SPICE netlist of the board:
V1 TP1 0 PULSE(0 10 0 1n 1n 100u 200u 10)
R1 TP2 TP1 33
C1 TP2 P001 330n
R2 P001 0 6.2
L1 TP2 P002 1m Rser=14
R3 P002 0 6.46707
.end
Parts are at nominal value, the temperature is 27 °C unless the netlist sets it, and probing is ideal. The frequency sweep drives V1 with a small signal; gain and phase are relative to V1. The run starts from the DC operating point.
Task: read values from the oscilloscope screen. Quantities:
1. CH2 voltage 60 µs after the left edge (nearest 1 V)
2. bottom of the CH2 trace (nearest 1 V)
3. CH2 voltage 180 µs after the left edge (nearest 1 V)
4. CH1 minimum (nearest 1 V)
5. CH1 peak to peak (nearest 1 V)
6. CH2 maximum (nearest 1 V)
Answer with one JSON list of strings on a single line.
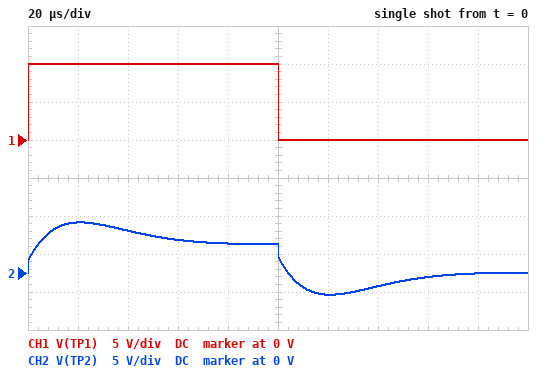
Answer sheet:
["4 V", "-3 V", "0 V", "0 V", "10 V", "7 V"]
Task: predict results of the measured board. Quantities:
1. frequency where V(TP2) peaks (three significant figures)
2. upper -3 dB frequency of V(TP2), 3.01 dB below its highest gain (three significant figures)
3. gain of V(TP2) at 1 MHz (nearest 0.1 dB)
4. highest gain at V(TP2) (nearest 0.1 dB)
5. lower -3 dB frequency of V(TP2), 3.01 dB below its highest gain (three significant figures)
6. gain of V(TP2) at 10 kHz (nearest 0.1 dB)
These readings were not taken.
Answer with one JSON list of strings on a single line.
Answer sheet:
["9.68 kHz", "21.0 kHz", "-16.0 dB", "-2.0 dB", "3.81 kHz", "-2.0 dB"]
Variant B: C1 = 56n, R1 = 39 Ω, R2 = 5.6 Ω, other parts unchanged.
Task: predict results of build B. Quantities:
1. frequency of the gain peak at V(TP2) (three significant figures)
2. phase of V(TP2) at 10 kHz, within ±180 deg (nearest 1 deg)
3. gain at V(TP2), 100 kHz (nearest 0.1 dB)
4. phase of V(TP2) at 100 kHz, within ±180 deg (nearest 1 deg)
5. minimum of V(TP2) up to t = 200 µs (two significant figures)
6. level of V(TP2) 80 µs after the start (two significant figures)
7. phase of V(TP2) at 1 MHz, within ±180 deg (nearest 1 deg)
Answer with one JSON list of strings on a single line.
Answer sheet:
["23.8 kHz", "20 deg", "-5.0 dB", "-45 deg", "-4.9 V", "3.5 V", "-23 deg"]
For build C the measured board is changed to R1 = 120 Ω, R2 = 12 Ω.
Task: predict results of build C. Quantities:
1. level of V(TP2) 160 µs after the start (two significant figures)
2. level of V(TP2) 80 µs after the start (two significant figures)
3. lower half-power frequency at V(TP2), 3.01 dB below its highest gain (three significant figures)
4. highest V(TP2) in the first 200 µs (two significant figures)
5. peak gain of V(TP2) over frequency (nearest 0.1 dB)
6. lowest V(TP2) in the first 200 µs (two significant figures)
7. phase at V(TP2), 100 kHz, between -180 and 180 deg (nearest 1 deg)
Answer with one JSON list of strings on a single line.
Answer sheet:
["-170 mV", "1.2 V", "5.31 kHz", "3.1 V", "-6.7 dB", "-1.7 V", "-19 deg"]
